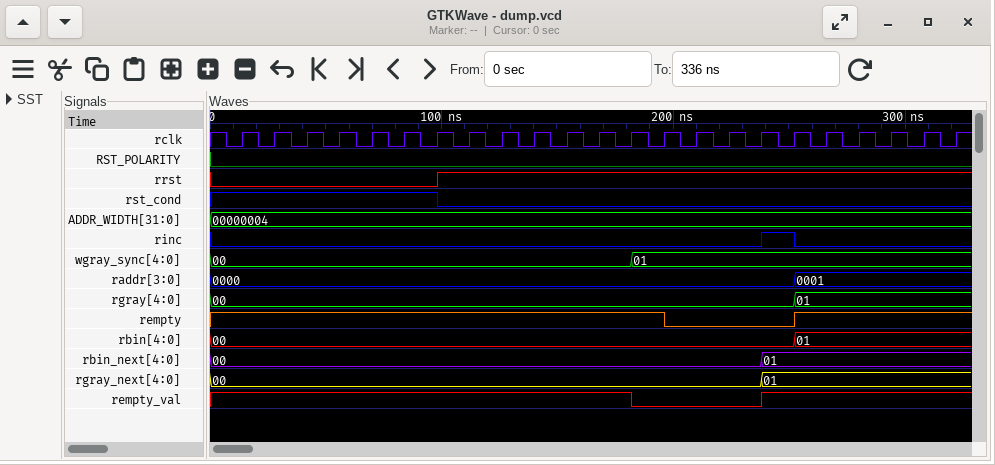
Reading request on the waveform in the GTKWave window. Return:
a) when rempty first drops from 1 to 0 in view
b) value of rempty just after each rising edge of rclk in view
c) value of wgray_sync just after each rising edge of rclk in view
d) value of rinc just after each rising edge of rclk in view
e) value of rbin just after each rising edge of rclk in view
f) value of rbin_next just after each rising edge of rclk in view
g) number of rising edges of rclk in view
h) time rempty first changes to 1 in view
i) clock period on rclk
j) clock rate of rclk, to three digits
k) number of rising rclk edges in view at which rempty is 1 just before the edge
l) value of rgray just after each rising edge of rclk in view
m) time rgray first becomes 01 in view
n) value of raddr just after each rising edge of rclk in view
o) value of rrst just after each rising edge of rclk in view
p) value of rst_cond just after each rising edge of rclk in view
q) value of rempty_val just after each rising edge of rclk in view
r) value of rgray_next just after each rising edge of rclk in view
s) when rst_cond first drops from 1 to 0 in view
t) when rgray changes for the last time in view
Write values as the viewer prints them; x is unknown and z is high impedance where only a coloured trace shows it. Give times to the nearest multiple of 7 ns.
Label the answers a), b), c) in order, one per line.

a) 196 ns
b) 1 1 1 1 1 1 1 1 1 1 1 1 1 0 0 0 0 1 1 1 1 1 1
c) 00, 00, 00, 00, 00, 00, 00, 00, 00, 00, 00, 00, 01, 01, 01, 01, 01, 01, 01, 01, 01, 01, 01
d) 0 0 0 0 0 0 0 0 0 0 0 0 0 0 0 0 1 0 0 0 0 0 0
e) 00, 00, 00, 00, 00, 00, 00, 00, 00, 00, 00, 00, 00, 00, 00, 00, 00, 01, 01, 01, 01, 01, 01
f) 00, 00, 00, 00, 00, 00, 00, 00, 00, 00, 00, 00, 00, 00, 00, 00, 01, 01, 01, 01, 01, 01, 01
g) 23
h) 252 ns
i) 14 ns
j) 71.4 MHz
k) 19
l) 00, 00, 00, 00, 00, 00, 00, 00, 00, 00, 00, 00, 00, 00, 00, 00, 00, 01, 01, 01, 01, 01, 01
m) 252 ns
n) 0000, 0000, 0000, 0000, 0000, 0000, 0000, 0000, 0000, 0000, 0000, 0000, 0000, 0000, 0000, 0000, 0000, 0001, 0001, 0001, 0001, 0001, 0001
o) 0 0 0 0 0 0 1 1 1 1 1 1 1 1 1 1 1 1 1 1 1 1 1
p) 1 1 1 1 1 1 0 0 0 0 0 0 0 0 0 0 0 0 0 0 0 0 0
q) 1 1 1 1 1 1 1 1 1 1 1 1 0 0 0 0 1 1 1 1 1 1 1
r) 00, 00, 00, 00, 00, 00, 00, 00, 00, 00, 00, 00, 00, 00, 00, 00, 01, 01, 01, 01, 01, 01, 01
s) 98 ns
t) 252 ns
